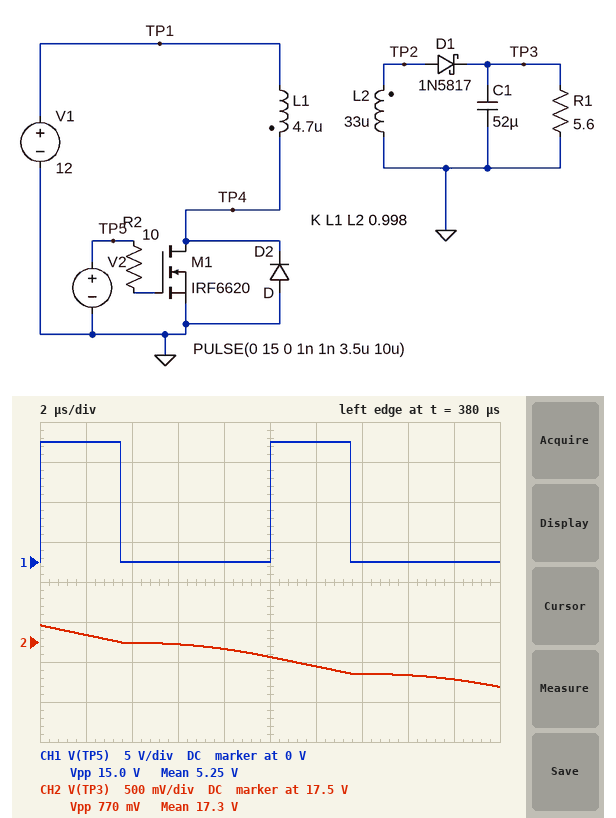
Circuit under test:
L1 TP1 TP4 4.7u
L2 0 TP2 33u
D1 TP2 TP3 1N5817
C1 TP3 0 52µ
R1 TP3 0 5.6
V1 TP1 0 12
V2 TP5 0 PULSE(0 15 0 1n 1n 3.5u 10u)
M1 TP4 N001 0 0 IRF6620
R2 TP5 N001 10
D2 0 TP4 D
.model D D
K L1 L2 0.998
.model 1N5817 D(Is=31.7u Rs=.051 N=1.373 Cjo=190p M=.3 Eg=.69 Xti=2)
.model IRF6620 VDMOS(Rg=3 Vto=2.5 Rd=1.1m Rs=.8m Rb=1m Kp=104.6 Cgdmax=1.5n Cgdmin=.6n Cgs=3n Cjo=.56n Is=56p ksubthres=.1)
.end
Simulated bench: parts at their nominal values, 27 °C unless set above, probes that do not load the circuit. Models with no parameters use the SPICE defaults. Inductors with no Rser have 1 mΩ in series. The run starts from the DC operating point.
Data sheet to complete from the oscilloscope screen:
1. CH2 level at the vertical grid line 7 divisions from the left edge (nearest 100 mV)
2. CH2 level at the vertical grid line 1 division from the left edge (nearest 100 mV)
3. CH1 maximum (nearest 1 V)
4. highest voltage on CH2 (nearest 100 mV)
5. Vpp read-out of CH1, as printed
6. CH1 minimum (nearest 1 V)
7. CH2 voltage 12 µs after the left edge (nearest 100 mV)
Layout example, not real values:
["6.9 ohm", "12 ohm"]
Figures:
["17.1 V", "17.6 V", "15 V", "17.7 V", "15.0 V", "0 V", "17.2 V"]
